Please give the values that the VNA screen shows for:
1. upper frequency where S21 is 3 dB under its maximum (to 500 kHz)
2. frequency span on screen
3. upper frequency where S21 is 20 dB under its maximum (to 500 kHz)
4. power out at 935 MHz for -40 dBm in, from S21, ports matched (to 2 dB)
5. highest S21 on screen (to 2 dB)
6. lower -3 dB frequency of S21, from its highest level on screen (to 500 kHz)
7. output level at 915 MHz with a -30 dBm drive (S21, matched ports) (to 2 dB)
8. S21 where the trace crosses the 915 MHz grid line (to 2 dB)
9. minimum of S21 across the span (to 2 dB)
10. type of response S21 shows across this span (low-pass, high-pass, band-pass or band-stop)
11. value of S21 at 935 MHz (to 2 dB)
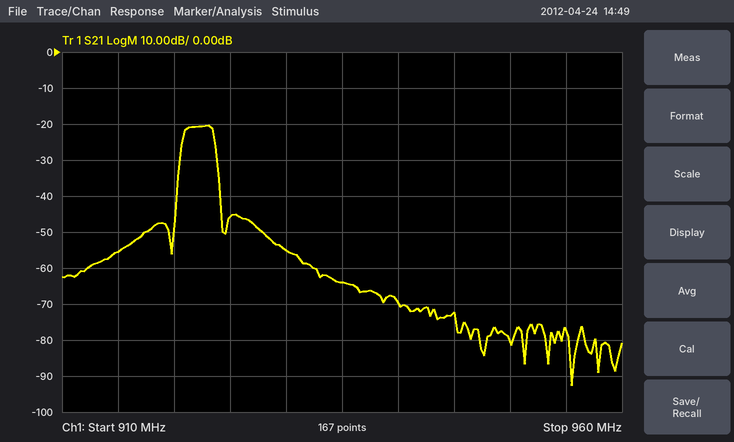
923.5 MHz
50 MHz
924.0 MHz
-104 dBm
-20 dB
921.0 MHz
-86 dBm
-56 dB
-92 dB
band-pass
-64 dB
